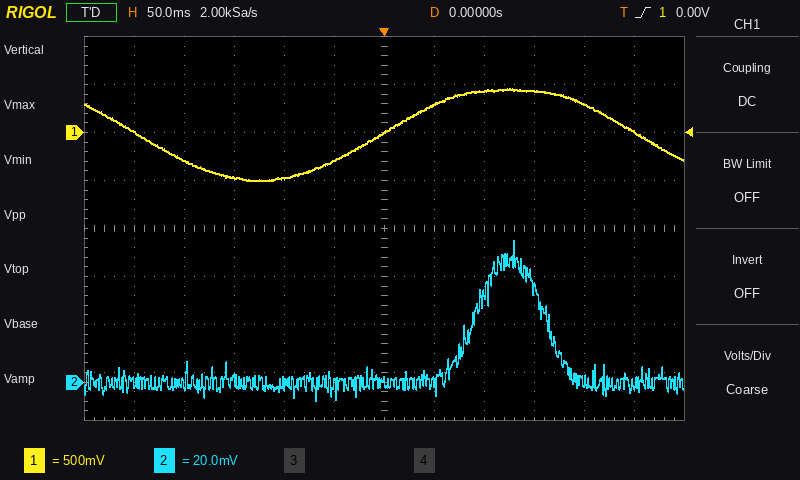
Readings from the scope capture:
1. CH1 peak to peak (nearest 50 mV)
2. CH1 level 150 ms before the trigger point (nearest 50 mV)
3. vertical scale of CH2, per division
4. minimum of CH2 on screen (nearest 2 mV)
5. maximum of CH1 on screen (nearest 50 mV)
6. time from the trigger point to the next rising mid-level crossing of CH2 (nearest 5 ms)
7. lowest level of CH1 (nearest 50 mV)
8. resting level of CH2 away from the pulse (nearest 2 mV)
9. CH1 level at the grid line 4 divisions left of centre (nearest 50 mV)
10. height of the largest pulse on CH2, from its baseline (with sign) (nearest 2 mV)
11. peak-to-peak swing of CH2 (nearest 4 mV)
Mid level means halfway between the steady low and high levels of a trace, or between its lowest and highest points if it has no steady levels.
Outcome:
950 mV
-450 mV
20 mV
-8 mV
450 mV
90 ms
-500 mV
0 mV
-300 mV
+58 mV
68 mV
